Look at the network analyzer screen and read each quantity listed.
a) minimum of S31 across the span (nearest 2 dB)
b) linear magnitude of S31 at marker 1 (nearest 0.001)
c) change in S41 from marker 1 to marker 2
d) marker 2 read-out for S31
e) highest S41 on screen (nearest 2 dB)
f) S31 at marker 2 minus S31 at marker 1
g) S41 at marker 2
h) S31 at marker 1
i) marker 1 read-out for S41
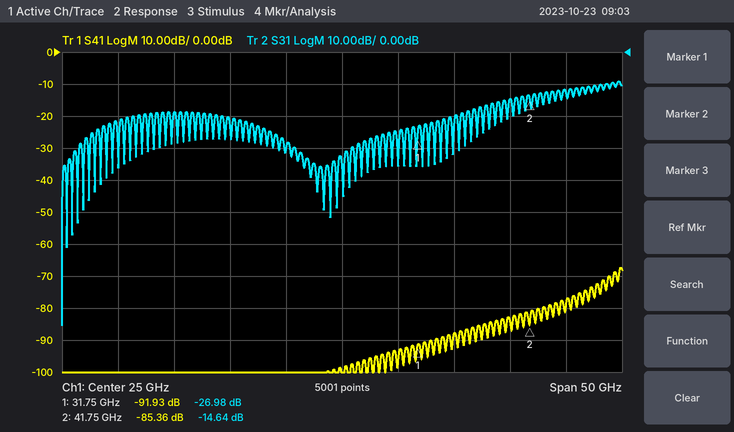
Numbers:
-86 dB
0.045
6.57 dB
-14.64 dB
-68 dB
12.34 dB
-85.36 dB
-26.98 dB
-91.93 dB
